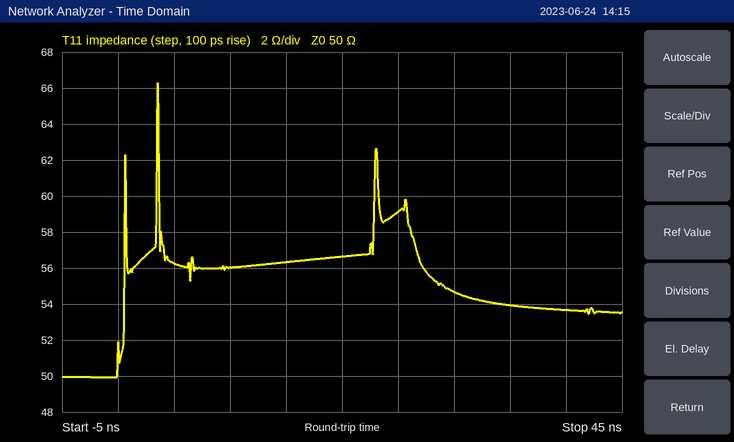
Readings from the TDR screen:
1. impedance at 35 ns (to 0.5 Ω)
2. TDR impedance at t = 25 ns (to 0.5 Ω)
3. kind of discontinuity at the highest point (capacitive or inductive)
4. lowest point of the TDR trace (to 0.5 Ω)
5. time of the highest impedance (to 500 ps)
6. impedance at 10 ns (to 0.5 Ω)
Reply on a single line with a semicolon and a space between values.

54.0 Ω; 59.0 Ω; inductive; 50.0 Ω; 3.5 ns; 56.0 Ω
